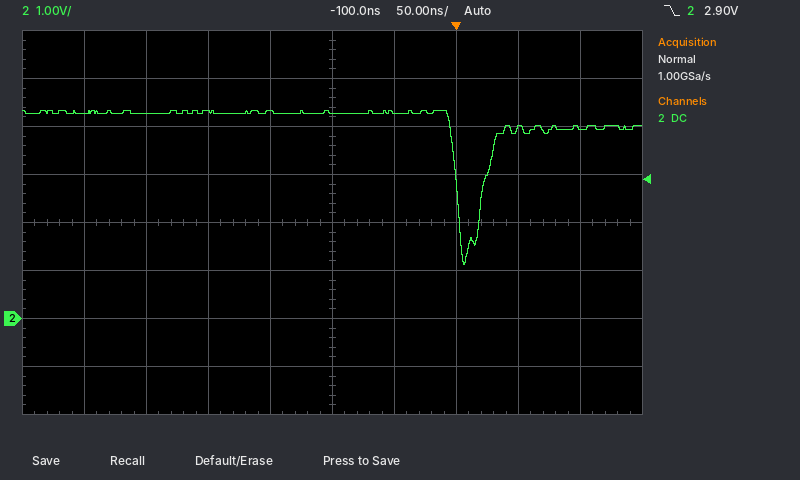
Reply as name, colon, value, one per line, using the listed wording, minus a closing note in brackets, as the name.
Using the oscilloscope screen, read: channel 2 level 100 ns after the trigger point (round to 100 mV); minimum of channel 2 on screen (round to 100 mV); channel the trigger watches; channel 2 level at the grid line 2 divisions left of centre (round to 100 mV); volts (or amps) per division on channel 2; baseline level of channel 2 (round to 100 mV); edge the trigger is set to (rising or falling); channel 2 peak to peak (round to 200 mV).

channel 2 level 100 ns after the trigger point: 4.0 V
minimum of channel 2 on screen: 1.1 V
channel the trigger watches: channel 2
channel 2 level at the grid line 2 divisions left of centre: 4.3 V
volts (or amps) per division on channel 2: 1 V
baseline level of channel 2: 4.3 V
edge the trigger is set to: falling
channel 2 peak to peak: 3.2 V
